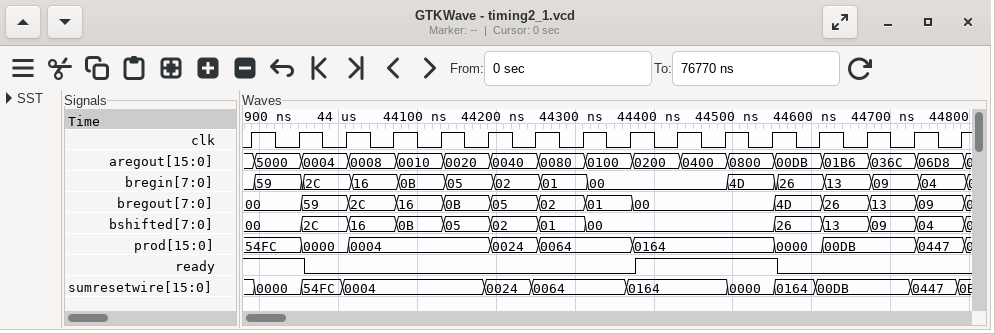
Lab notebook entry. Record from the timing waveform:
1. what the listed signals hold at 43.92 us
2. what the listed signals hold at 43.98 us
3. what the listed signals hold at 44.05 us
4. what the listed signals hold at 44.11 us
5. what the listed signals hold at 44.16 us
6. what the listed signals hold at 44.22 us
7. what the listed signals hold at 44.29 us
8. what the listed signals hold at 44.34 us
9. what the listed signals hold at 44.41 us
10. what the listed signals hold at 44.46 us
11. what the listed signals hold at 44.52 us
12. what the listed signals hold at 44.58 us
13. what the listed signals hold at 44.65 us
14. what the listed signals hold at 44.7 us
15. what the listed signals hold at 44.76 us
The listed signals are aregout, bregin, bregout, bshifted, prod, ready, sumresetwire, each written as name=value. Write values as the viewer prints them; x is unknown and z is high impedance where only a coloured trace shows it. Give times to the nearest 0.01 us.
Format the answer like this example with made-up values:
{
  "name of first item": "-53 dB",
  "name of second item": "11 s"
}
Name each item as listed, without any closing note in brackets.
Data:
{
  "what the listed signals hold at 43.92 us": "aregout=5000, bregin=59, bregout=00, bshifted=00, prod=54FC, ready=1, sumresetwire=0000",
  "what the listed signals hold at 43.98 us": "aregout=0004, bregin=2C, bregout=59, bshifted=2C, prod=0000, ready=0, sumresetwire=54FC",
  "what the listed signals hold at 44.05 us": "aregout=0008, bregin=16, bregout=2C, bshifted=16, prod=0004, ready=0, sumresetwire=0004",
  "what the listed signals hold at 44.11 us": "aregout=0010, bregin=0B, bregout=16, bshifted=0B, prod=0004, ready=0, sumresetwire=0004",
  "what the listed signals hold at 44.16 us": "aregout=0020, bregin=05, bregout=0B, bshifted=05, prod=0004, ready=0, sumresetwire=0004",
  "what the listed signals hold at 44.22 us": "aregout=0040, bregin=02, bregout=05, bshifted=02, prod=0024, ready=0, sumresetwire=0024",
  "what the listed signals hold at 44.29 us": "aregout=0080, bregin=01, bregout=02, bshifted=01, prod=0064, ready=0, sumresetwire=0064",
  "what the listed signals hold at 44.34 us": "aregout=0100, bregin=00, bregout=01, bshifted=00, prod=0064, ready=0, sumresetwire=0064",
  "what the listed signals hold at 44.41 us": "aregout=0200, bregin=00, bregout=00, bshifted=00, prod=0164, ready=1, sumresetwire=0164",
  "what the listed signals hold at 44.46 us": "aregout=0400, bregin=00, bregout=00, bshifted=00, prod=0164, ready=1, sumresetwire=0164",
  "what the listed signals hold at 44.52 us": "aregout=0800, bregin=4D, bregout=00, bshifted=00, prod=0164, ready=1, sumresetwire=0000",
  "what the listed signals hold at 44.58 us": "aregout=00DB, bregin=26, bregout=4D, bshifted=26, prod=0000, ready=0, sumresetwire=0164",
  "what the listed signals hold at 44.65 us": "aregout=01B6, bregin=13, bregout=26, bshifted=13, prod=00DB, ready=0, sumresetwire=00DB",
  "what the listed signals hold at 44.7 us": "aregout=036C, bregin=09, bregout=13, bshifted=09, prod=00DB, ready=0, sumresetwire=00DB",
  "what the listed signals hold at 44.76 us": "aregout=06D8, bregin=04, bregout=09, bshifted=04, prod=0447, ready=0, sumresetwire=0447"
}
